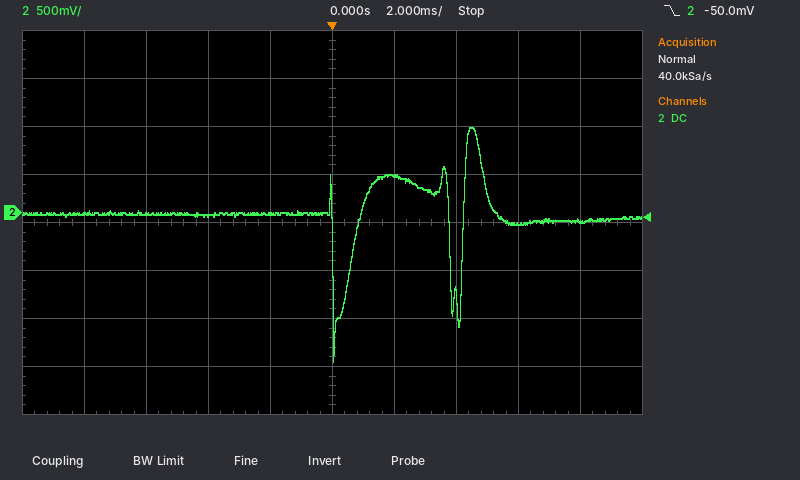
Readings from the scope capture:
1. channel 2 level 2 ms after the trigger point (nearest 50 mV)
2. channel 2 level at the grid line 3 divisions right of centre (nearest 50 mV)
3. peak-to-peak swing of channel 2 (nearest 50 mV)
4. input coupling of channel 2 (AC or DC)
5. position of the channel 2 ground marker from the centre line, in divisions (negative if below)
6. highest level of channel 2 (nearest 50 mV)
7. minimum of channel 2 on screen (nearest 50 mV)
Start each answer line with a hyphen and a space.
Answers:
- 400 mV
- -100 mV
- 2.45 V
- DC
- +0.2 div
- 900 mV
- -1.55 V
